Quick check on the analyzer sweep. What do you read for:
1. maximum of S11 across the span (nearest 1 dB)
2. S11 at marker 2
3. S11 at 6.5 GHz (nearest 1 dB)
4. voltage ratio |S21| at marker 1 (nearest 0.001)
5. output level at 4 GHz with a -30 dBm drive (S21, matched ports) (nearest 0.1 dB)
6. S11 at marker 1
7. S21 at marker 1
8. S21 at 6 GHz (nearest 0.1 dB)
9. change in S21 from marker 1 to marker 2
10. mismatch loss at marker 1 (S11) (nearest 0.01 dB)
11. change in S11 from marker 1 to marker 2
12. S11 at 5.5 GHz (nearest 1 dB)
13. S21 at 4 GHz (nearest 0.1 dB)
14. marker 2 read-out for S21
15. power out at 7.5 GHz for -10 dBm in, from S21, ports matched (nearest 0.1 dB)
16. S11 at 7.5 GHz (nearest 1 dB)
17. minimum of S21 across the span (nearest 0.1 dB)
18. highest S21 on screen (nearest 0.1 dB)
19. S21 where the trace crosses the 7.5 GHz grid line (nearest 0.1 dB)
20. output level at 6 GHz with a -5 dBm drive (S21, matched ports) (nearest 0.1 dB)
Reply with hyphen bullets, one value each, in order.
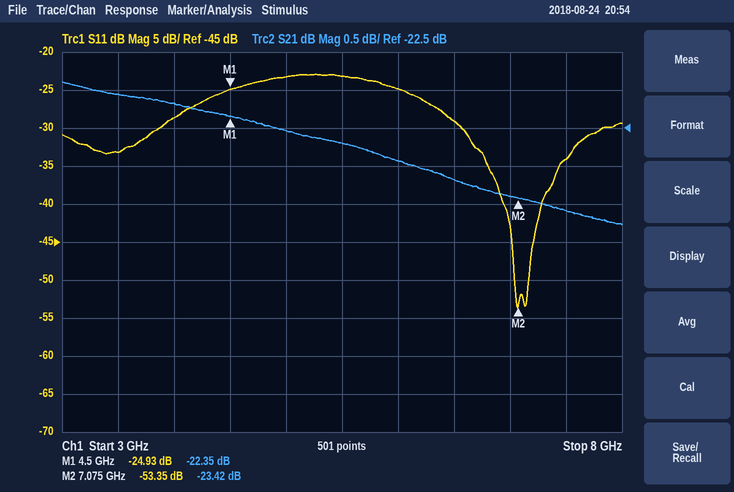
- -23 dB
- -53.35 dB
- -29 dB
- 0.076
- -52.2 dBm
- -24.93 dB
- -22.35 dB
- -22.9 dB
- -1.07 dB
- 0.01 dB
- -28.42 dB
- -23 dB
- -22.2 dB
- -23.42 dB
- -33.6 dBm
- -34 dB
- -23.8 dB
- -21.9 dB
- -23.6 dB
- -27.9 dBm
